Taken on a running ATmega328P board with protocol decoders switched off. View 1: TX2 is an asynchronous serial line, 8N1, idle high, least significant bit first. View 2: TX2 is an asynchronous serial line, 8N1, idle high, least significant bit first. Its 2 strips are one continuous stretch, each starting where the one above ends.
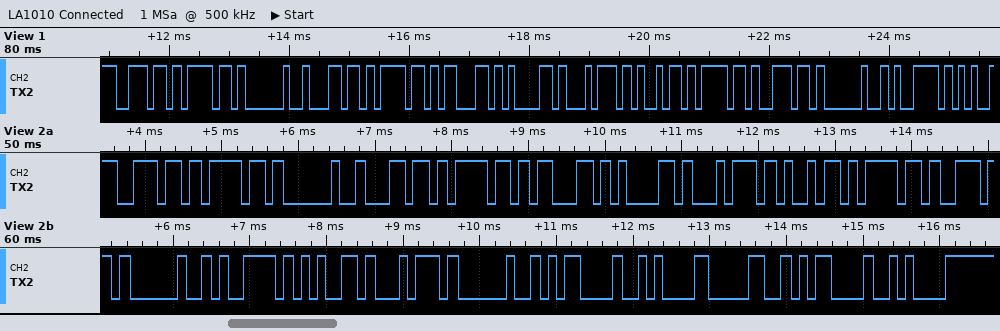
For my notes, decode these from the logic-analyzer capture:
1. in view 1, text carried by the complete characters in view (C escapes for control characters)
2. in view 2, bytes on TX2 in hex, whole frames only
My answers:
"no location y"
0x6E 0x6F 0x20 0x6C 0x6F 0x63 0x61 0x74 0x69 0x6F 0x6E 0x20 0x79 0x65 0x74 0x20 0x0D 0x0A 0x30 0x0D 0x0A
